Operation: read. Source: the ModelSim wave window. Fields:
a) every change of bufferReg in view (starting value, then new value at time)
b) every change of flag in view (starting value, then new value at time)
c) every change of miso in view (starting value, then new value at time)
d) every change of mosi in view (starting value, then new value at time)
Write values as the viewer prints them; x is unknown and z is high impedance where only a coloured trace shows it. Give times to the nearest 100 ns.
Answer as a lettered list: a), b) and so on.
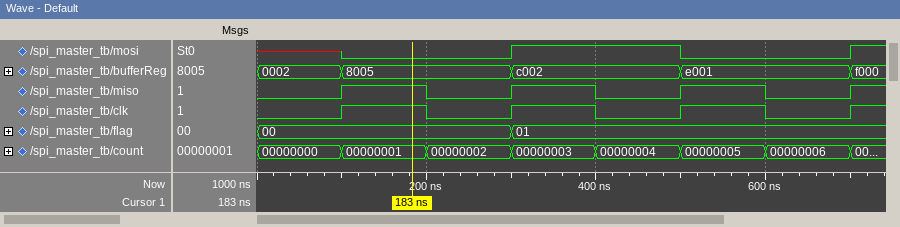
a) 0002, 8005 at 100 ns, c002 at 300 ns, e001 at 500 ns, f000 at 700 ns
b) 00, 01 at 300 ns
c) 0, 1 at 100 ns, 0 at 200 ns, 1 at 300 ns, 0 at 400 ns, 1 at 500 ns, 0 at 600 ns, 1 at 700 ns
d) x, 0 at 100 ns, 1 at 300 ns, 0 at 500 ns, 1 at 700 ns
